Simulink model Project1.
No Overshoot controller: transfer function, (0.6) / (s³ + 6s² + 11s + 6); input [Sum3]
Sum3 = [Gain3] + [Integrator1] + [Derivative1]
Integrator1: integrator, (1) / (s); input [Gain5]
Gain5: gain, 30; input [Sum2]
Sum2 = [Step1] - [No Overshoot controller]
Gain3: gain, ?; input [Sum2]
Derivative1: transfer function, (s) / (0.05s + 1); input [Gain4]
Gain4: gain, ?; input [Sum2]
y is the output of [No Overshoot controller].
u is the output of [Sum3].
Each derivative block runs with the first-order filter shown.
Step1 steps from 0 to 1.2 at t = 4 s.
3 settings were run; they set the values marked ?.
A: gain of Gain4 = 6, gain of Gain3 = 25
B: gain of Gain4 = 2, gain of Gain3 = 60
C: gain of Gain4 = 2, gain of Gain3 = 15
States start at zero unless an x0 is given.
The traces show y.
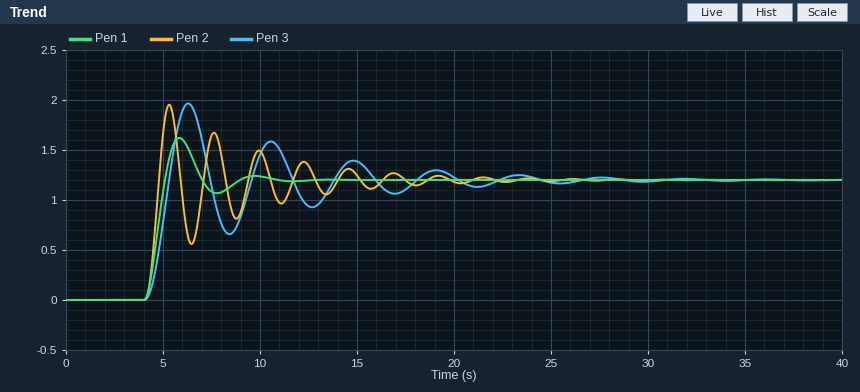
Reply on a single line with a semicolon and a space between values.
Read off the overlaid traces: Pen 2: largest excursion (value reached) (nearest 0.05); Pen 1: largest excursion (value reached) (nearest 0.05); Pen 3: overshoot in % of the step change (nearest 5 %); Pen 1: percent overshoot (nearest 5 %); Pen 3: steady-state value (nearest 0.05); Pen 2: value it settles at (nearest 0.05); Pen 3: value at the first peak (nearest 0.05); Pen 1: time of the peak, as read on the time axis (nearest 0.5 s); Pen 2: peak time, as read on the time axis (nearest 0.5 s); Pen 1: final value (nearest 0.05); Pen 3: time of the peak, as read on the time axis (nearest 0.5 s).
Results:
1.95; 1.60; 65 %; 35 %; 1.20; 1.20; 1.95; 6.0 s; 5.5 s; 1.20; 6.5 s
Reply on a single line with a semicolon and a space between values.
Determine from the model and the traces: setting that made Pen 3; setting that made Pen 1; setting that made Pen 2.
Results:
C; A; B
